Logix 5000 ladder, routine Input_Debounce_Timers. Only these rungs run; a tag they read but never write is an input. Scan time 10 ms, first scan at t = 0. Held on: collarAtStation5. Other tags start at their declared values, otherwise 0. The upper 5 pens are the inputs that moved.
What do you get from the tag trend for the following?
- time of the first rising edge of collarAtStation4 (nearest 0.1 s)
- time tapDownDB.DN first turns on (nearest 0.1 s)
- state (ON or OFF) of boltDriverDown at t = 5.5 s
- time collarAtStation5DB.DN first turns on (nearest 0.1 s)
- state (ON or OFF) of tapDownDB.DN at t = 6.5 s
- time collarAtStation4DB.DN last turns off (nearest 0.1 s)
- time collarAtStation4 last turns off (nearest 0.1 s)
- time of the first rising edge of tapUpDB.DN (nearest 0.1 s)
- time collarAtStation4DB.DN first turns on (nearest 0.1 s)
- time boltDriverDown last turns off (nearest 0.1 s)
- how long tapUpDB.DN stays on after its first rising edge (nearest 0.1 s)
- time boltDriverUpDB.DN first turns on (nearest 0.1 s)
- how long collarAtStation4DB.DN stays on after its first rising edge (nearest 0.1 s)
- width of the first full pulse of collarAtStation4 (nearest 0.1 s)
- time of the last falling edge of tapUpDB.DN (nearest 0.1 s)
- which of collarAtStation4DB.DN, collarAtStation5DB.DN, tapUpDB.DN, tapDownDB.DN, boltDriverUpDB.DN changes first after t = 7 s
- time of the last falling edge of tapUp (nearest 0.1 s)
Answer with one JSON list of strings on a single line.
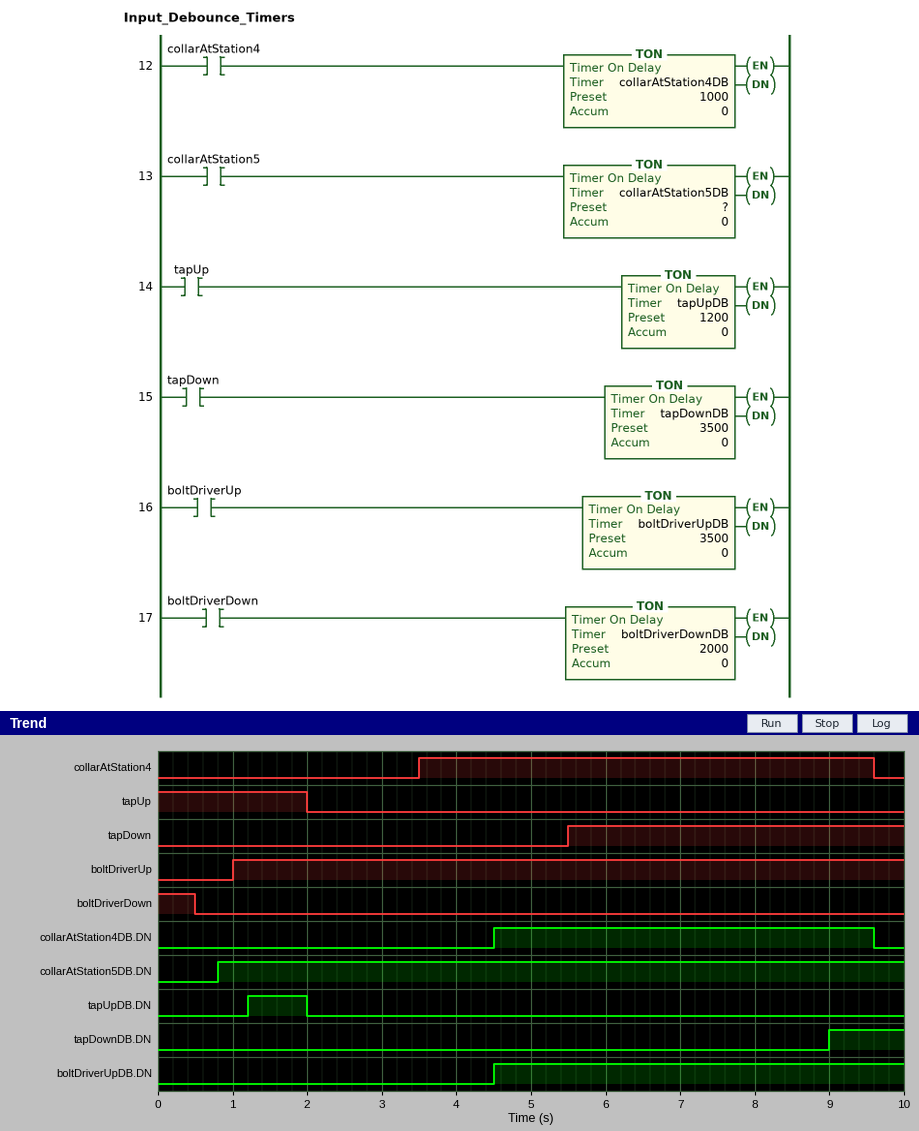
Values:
["3.5 s", "9.0 s", "OFF", "0.8 s", "OFF", "9.6 s", "9.6 s", "1.2 s", "4.5 s", "0.5 s", "0.8 s", "4.5 s", "5.1 s", "6.1 s", "2.0 s", "tapDownDB.DN", "2.0 s"]
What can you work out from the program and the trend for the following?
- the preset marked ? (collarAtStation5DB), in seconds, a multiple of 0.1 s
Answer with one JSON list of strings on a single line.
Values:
["0.8 s"]
